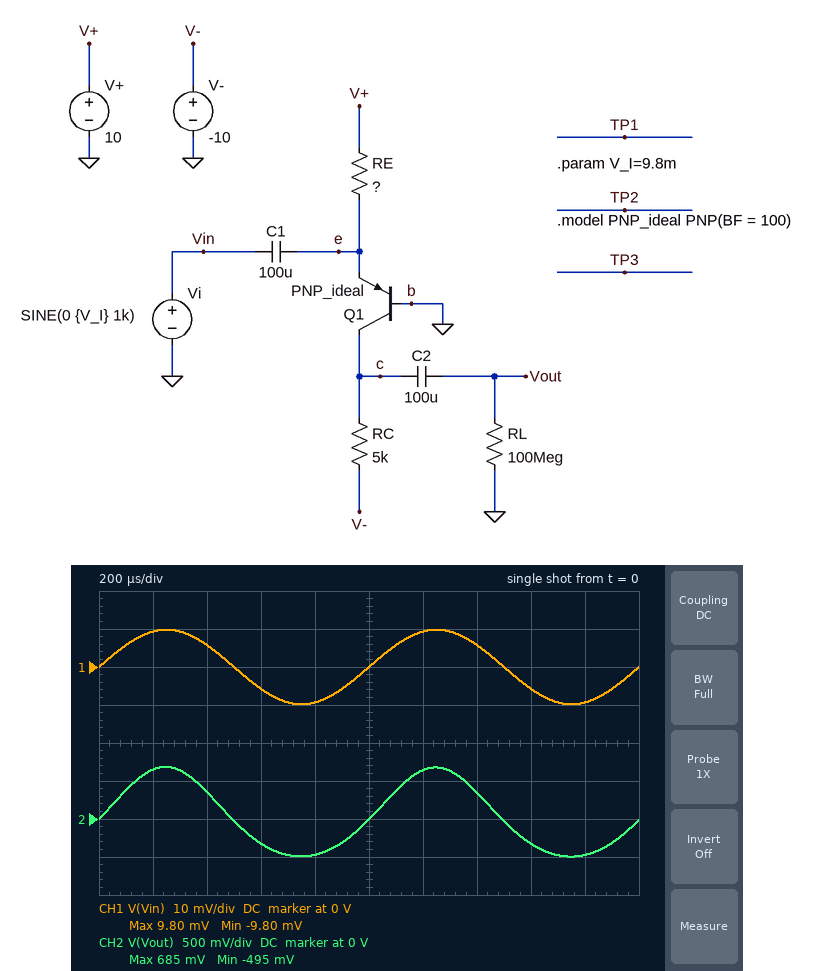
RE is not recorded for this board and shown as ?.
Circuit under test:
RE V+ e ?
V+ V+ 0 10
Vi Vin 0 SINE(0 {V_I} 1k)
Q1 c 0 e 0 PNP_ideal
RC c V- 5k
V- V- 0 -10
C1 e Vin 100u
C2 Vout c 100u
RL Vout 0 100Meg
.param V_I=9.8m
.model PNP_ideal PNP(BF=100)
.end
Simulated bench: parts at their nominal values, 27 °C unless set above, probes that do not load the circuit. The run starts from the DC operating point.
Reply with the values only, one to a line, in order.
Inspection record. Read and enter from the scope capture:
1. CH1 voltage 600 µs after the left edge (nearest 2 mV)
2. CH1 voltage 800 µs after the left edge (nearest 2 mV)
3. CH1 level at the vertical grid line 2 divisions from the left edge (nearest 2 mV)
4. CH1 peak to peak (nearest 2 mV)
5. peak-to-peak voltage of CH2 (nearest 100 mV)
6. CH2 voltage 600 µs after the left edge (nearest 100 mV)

-6 mV
-10 mV
6 mV
20 mV
1.2 V
-300 mV
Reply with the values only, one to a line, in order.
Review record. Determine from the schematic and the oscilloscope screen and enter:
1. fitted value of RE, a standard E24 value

30 kΩ
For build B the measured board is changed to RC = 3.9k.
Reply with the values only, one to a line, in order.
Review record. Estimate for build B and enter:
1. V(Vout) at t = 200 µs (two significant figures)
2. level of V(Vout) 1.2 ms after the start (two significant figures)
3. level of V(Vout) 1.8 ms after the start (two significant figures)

510 mV
500 mV
-370 mV
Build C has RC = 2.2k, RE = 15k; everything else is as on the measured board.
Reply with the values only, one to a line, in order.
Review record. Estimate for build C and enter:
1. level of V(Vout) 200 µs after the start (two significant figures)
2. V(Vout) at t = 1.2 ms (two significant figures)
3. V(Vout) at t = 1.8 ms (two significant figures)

560 mV
550 mV
-420 mV
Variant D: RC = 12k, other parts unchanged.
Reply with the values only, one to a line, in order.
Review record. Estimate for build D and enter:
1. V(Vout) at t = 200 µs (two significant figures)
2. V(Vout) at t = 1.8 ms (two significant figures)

1.6 V
-1.1 V
